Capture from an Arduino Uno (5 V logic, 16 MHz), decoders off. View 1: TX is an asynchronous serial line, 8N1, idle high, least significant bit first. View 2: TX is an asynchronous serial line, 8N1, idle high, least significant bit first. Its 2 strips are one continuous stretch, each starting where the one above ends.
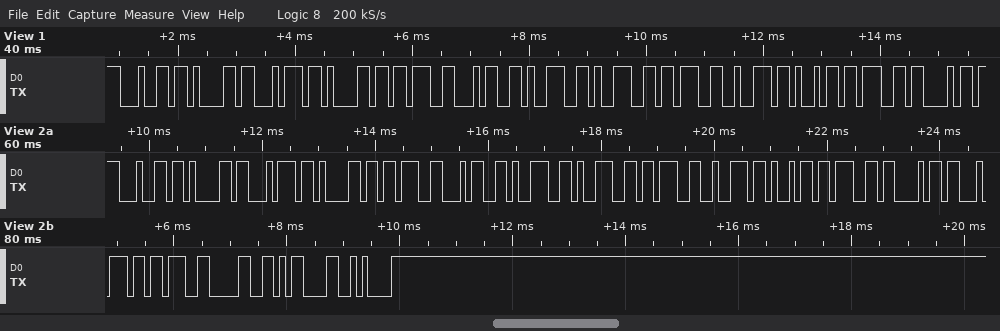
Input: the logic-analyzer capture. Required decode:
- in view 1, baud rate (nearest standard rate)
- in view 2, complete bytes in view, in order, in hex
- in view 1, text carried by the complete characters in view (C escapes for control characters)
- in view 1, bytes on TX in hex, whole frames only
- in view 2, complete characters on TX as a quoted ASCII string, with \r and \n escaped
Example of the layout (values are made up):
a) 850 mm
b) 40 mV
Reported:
a) 9600 baud
b) 64 61 74 61 3B 34 39 39 3B 72 69 67 68 74 3B 30 0D 0A
c) "data;499;righ"
d) 64 61 74 61 3B 34 39 39 3B 72 69 67 68
e) "data;499;right;0\r\n"
